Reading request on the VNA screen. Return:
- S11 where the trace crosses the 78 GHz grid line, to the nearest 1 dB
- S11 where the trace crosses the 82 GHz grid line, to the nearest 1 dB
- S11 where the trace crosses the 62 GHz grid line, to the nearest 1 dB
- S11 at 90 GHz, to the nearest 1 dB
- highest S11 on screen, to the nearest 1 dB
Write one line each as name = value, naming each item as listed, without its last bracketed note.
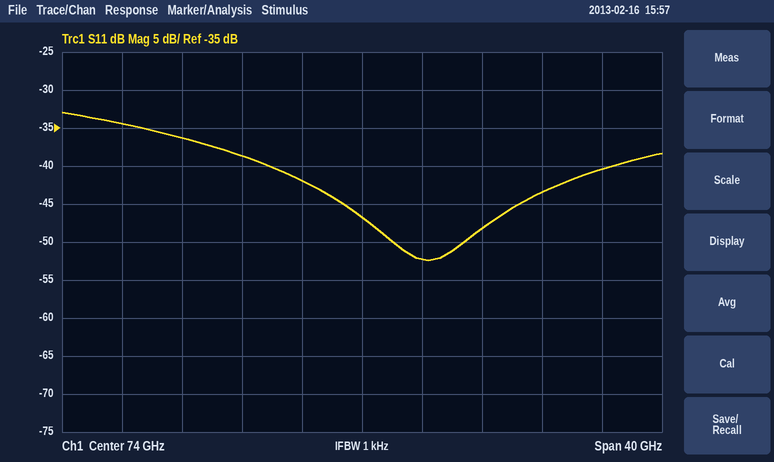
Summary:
S11 where the trace crosses the 78 GHz grid line, to the nearest 1 dB = -52 dB
S11 where the trace crosses the 82 GHz grid line, to the nearest 1 dB = -48 dB
S11 where the trace crosses the 62 GHz grid line, to the nearest 1 dB = -36 dB
S11 at 90 GHz, to the nearest 1 dB = -40 dB
highest S11 on screen, to the nearest 1 dB = -33 dB
